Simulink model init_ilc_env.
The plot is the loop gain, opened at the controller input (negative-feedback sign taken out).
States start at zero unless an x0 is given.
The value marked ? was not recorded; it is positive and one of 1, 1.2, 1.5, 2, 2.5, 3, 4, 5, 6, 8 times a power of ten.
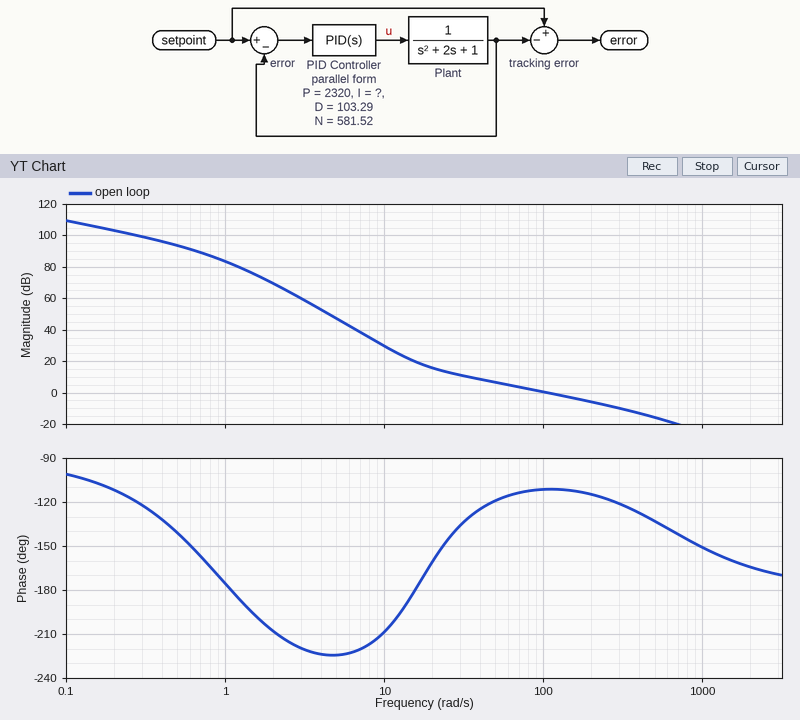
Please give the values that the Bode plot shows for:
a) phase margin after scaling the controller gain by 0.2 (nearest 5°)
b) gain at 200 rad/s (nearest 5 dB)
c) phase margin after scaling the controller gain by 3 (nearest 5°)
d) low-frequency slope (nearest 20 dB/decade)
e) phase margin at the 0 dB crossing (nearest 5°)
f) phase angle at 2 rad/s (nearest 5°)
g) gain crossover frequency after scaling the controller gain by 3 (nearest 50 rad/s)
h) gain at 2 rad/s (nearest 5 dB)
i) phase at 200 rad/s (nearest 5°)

30°
-5 dB
60°
-20 dB/decade
70°
-210°
300 rad/s
70 dB
-115°
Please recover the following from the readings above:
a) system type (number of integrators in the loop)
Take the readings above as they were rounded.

1
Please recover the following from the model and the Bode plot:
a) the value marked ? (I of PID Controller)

30000
